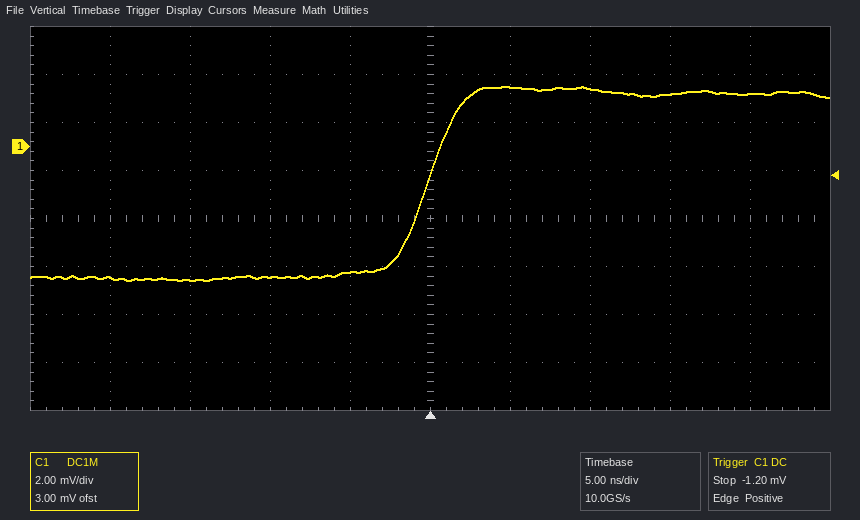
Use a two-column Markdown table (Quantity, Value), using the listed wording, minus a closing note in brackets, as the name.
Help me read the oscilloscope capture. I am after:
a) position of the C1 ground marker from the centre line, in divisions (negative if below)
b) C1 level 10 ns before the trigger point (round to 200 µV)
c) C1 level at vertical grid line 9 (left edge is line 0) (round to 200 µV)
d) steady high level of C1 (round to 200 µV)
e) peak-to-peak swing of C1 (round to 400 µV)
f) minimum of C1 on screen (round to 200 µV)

| Quantity | Value |
|---|---|
| position of the C1 ground marker from the centre line, in divisions | +1.5 div |
| C1 level 10 ns before the trigger point | -5.4 mV |
| C1 level at vertical grid line 9 (left edge is line 0) | 2.2 mV |
| steady high level of C1 | 2.2 mV |
| peak-to-peak swing of C1 | 8.0 mV |
| minimum of C1 on screen | -5.6 mV |
